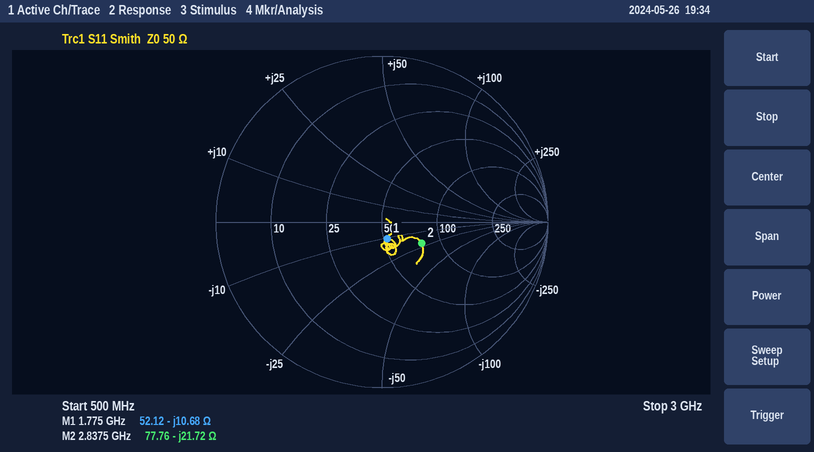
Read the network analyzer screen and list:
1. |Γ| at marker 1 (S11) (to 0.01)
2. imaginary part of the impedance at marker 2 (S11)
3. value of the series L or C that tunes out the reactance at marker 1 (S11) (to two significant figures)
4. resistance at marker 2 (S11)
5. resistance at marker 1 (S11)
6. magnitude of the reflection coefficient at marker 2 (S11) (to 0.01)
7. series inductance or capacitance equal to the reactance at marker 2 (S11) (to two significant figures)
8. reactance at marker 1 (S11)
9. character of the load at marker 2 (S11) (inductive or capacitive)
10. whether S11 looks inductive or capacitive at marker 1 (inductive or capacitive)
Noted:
0.11
-21.72 Ω
960 pH
77.76 Ω
52.12 Ω
0.27
2.6 pF
-10.68 Ω
capacitive
capacitive
